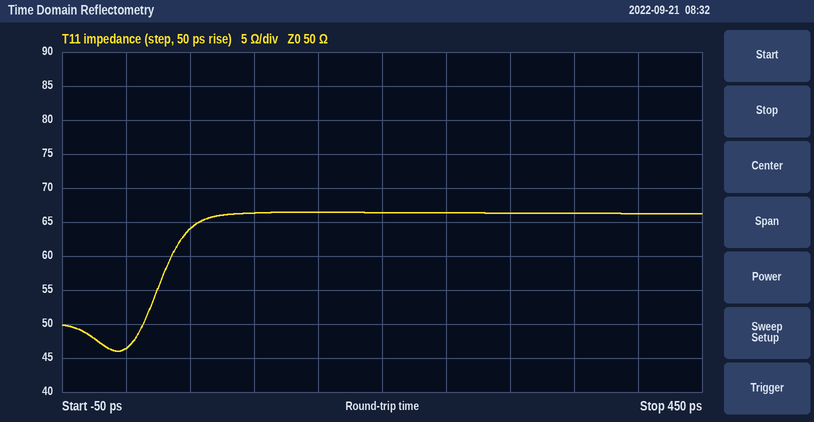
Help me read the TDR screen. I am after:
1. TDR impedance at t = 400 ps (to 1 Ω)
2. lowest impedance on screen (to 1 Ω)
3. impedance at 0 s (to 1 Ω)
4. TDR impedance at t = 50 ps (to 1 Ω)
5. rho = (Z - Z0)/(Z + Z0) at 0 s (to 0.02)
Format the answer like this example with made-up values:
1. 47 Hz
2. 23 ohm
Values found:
1. 66 Ω
2. 46 Ω
3. 46 Ω
4. 64 Ω
5. -0.04
